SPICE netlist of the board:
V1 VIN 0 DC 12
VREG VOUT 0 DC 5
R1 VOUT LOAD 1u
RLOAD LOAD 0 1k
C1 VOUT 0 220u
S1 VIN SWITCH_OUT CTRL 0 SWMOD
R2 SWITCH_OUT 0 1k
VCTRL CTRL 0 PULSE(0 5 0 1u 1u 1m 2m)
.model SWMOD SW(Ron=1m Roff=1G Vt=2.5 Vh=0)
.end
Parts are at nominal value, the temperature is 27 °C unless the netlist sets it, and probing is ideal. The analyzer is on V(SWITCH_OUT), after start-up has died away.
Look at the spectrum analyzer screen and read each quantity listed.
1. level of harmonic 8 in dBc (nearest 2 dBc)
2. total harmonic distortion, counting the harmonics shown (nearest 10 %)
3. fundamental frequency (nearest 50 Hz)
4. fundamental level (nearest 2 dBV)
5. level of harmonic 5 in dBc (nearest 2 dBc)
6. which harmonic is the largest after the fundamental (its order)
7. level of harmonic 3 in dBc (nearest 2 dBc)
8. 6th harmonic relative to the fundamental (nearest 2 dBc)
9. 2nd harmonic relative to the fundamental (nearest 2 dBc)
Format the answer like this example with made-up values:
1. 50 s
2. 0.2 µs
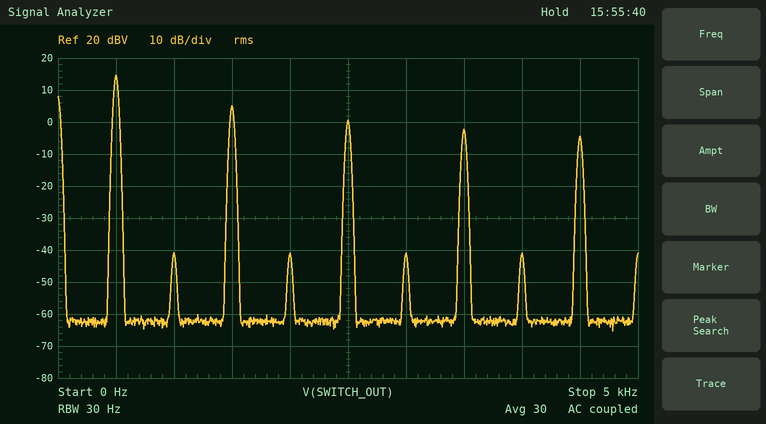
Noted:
1. -56 dBc
2. 40 %
3. 500 Hz
4. 14 dBV
5. -14 dBc
6. 3
7. -10 dBc
8. -56 dBc
9. -56 dBc
